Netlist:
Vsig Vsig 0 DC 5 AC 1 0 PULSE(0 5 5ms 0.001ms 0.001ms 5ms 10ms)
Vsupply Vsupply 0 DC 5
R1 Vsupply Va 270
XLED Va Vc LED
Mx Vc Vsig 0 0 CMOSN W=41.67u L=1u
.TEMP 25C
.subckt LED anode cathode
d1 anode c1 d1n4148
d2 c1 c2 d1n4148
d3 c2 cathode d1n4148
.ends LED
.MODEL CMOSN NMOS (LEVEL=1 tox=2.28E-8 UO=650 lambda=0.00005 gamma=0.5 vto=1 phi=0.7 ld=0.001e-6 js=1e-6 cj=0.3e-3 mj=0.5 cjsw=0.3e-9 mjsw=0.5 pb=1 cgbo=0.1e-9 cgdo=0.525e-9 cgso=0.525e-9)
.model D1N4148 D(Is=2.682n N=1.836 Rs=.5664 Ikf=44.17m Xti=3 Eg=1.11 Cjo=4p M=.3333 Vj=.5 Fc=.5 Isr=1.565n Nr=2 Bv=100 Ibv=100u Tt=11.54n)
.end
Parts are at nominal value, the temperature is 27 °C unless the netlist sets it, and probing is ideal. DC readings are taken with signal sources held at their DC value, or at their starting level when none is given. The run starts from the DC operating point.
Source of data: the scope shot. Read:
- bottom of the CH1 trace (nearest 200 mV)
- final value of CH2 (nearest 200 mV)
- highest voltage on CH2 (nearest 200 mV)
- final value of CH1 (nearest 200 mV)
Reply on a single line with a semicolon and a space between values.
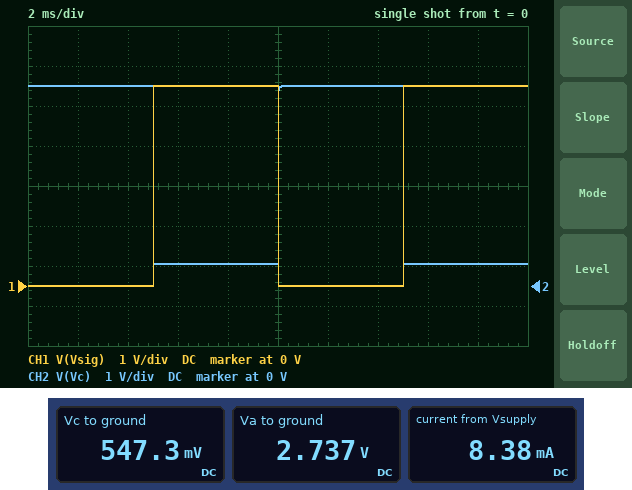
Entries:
0 V; 600 mV; 5.0 V; 5.0 V
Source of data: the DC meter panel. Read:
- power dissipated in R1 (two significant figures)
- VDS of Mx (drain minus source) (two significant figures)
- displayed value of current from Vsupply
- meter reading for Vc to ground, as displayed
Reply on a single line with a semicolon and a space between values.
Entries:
19 mW; 550 mV; 8.38 mA; 547.3 mV
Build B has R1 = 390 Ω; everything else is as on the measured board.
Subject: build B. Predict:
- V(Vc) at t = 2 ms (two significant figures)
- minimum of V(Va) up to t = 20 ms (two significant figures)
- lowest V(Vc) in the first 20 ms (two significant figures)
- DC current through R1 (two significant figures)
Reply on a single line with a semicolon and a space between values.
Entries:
5.0 V; 2.5 V; 400 mV; 6.3 mA
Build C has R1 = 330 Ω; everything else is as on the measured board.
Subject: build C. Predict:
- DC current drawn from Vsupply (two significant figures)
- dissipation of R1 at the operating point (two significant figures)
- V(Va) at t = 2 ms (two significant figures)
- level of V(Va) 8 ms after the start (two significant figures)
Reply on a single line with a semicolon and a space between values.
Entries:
7.2 mA; 17 mW; 5.0 V; 2.6 V
